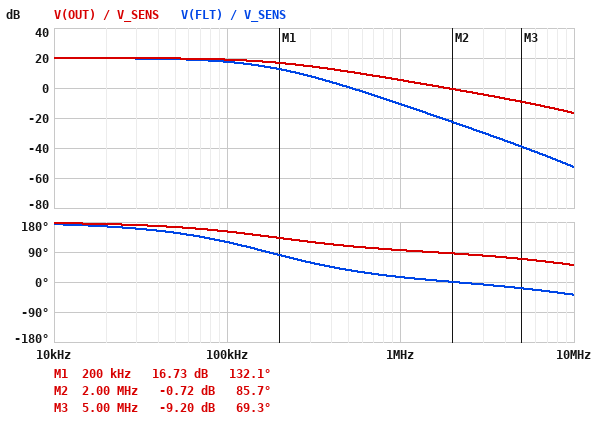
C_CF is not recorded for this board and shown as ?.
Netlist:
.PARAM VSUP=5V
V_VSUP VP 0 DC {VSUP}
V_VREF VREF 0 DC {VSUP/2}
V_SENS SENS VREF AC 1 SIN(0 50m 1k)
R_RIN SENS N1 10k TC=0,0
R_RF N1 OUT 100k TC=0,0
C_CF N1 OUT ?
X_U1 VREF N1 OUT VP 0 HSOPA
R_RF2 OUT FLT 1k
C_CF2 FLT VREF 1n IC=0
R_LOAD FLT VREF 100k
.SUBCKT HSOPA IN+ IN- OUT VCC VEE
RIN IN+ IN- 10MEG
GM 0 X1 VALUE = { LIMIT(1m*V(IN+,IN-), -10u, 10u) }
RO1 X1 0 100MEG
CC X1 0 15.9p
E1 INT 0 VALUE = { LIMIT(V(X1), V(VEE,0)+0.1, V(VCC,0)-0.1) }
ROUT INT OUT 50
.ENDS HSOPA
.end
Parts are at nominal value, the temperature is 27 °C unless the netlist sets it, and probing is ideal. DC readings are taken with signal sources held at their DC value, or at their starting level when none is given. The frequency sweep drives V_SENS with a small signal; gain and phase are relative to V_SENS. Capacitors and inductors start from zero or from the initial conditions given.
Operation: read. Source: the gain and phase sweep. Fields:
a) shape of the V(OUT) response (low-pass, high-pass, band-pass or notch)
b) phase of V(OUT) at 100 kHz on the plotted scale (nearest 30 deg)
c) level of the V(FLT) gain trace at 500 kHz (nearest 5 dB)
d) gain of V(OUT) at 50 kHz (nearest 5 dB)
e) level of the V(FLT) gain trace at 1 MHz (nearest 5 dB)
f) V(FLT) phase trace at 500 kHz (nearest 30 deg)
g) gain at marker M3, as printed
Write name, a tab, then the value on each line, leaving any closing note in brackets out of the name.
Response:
shape of the V(OUT) response	low-pass
phase of V(OUT) at 100 kHz on the plotted scale	150 deg
level of the V(FLT) gain trace at 500 kHz	0 dB
gain of V(OUT) at 50 kHz	20 dB
level of the V(FLT) gain trace at 1 MHz	-10 dB
V(FLT) phase trace at 500 kHz	30 deg
gain at marker M3, as printed	-9.20 dB
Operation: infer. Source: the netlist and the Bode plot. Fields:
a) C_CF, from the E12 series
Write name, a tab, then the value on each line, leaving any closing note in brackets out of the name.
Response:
C_CF, from the E12 series	6.8 pF
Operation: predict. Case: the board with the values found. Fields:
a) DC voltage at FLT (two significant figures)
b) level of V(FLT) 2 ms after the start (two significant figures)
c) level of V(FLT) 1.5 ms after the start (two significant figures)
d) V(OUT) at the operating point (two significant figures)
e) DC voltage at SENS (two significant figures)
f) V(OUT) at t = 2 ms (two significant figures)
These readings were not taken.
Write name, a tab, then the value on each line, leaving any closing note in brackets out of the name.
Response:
DC voltage at FLT	2.5 V
level of V(FLT) 2 ms after the start	2.5 V
level of V(FLT) 1.5 ms after the start	2.5 V
V(OUT) at the operating point	2.5 V
DC voltage at SENS	2.5 V
V(OUT) at t = 2 ms	2.5 V
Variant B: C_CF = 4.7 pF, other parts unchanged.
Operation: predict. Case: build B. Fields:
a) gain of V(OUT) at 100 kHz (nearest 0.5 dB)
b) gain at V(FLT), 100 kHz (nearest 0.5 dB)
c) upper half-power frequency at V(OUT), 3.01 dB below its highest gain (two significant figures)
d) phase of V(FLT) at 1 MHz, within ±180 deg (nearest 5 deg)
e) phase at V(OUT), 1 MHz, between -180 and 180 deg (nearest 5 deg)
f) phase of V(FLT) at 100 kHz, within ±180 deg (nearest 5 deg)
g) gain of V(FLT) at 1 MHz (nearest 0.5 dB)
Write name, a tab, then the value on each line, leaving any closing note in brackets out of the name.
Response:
gain of V(OUT) at 100 kHz	19.5 dB
gain at V(FLT), 100 kHz	18.0 dB
upper half-power frequency at V(OUT), 3.01 dB below its highest gain	250 kHz
phase of V(FLT) at 1 MHz, within ±180 deg	20 deg
phase at V(OUT), 1 MHz, between -180 and 180 deg	100 deg
phase of V(FLT) at 100 kHz, within ±180 deg	125 deg
gain of V(FLT) at 1 MHz	-8.5 dB
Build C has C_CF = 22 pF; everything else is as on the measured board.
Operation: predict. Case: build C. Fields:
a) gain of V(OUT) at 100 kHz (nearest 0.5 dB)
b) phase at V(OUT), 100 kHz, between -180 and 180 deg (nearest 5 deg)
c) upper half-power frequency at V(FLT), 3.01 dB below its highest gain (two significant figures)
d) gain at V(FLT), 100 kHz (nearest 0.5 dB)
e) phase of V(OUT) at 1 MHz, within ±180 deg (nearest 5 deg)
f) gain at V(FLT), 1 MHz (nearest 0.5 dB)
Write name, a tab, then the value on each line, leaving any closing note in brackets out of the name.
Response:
gain of V(OUT) at 100 kHz	15.0 dB
phase at V(OUT), 100 kHz, between -180 and 180 deg	125 deg
upper half-power frequency at V(FLT), 3.01 dB below its highest gain	59 kHz
gain at V(FLT), 100 kHz	13.5 dB
phase of V(OUT) at 1 MHz, within ±180 deg	90 deg
gain at V(FLT), 1 MHz	-19.5 dB
